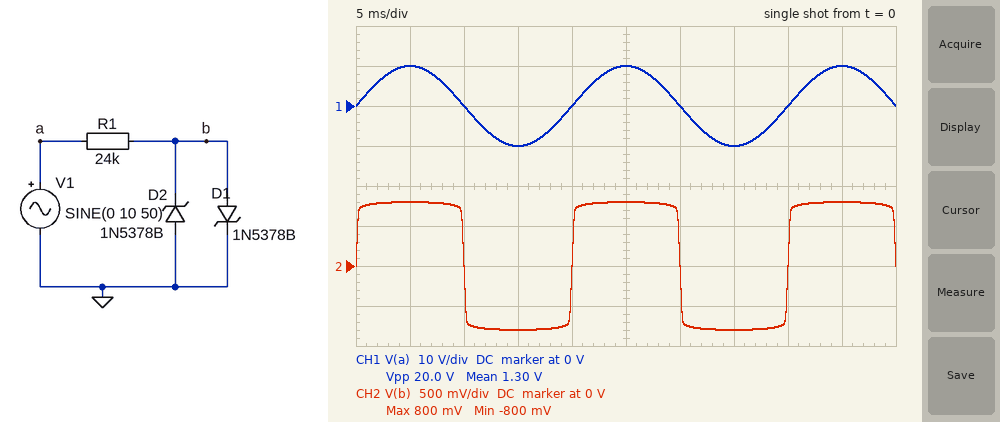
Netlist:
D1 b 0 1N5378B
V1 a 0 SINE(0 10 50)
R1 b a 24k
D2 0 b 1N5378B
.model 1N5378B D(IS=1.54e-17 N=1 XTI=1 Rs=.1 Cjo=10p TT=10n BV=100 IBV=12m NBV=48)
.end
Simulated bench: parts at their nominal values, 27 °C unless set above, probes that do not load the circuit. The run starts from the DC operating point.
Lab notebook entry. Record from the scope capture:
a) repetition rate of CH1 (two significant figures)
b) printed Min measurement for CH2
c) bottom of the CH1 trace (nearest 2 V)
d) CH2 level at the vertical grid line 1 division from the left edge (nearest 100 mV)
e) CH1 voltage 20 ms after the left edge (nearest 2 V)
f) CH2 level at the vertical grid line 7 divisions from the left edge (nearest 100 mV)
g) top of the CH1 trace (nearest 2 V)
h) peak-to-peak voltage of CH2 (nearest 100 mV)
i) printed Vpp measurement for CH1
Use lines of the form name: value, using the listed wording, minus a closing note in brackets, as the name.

repetition rate of CH1: 50 Hz
printed Min measurement for CH2: -800 mV
bottom of the CH1 trace: -10 V
CH2 level at the vertical grid line 1 division from the left edge: 800 mV
CH1 voltage 20 ms after the left edge: 0 V
CH2 level at the vertical grid line 7 divisions from the left edge: -800 mV
top of the CH1 trace: 10 V
peak-to-peak voltage of CH2: 1.6 V
printed Vpp measurement for CH1: 20.0 V
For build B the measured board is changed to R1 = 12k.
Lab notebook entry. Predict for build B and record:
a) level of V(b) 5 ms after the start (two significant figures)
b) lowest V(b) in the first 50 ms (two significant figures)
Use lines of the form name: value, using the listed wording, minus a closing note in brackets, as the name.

level of V(b) 5 ms after the start: 820 mV
lowest V(b) in the first 50 ms: -820 mV
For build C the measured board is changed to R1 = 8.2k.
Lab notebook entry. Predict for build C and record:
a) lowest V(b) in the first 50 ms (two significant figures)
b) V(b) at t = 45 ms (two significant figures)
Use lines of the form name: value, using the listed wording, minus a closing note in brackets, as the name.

lowest V(b) in the first 50 ms: -830 mV
V(b) at t = 45 ms: 830 mV
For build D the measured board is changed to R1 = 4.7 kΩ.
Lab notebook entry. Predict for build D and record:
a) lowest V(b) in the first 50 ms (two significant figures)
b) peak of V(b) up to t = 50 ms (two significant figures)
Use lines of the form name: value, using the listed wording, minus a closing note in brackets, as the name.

lowest V(b) in the first 50 ms: -840 mV
peak of V(b) up to t = 50 ms: 840 mV
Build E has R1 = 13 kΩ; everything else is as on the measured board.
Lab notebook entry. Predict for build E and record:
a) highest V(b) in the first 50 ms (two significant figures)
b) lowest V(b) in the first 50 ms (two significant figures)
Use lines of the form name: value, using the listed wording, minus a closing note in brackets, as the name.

highest V(b) in the first 50 ms: 810 mV
lowest V(b) in the first 50 ms: -810 mV
